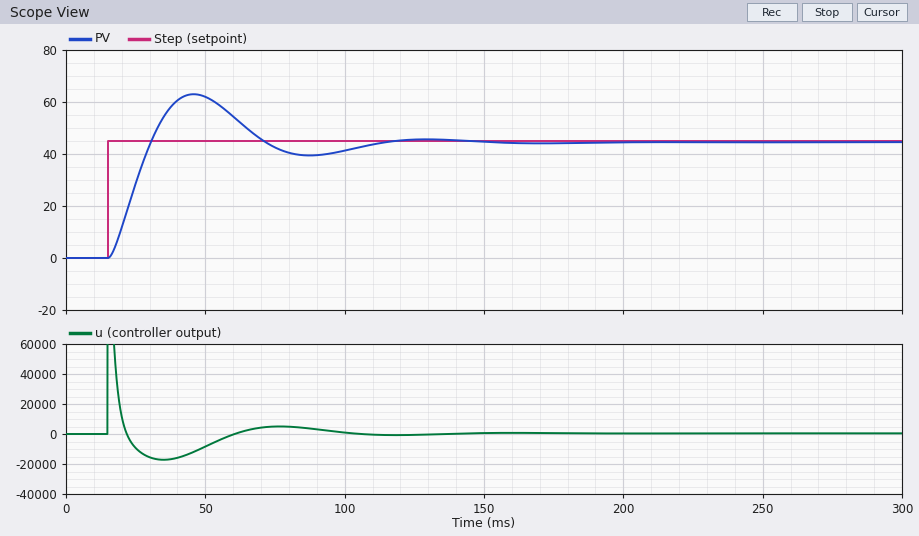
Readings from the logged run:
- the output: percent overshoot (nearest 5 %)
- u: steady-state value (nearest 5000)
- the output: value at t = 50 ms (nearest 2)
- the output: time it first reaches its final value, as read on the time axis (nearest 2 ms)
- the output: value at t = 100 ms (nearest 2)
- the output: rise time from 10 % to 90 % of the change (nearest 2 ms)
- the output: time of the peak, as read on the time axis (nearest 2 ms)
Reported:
40 %
0
62
30 ms
42
12 ms
46 ms
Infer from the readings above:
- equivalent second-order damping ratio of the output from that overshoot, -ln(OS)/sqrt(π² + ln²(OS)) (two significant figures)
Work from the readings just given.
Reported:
0.28
